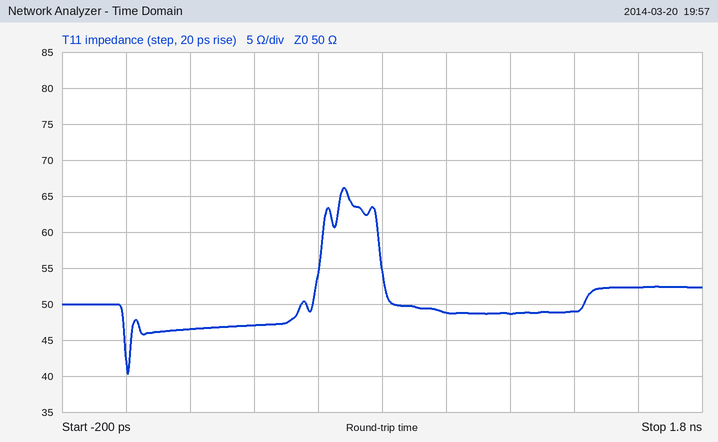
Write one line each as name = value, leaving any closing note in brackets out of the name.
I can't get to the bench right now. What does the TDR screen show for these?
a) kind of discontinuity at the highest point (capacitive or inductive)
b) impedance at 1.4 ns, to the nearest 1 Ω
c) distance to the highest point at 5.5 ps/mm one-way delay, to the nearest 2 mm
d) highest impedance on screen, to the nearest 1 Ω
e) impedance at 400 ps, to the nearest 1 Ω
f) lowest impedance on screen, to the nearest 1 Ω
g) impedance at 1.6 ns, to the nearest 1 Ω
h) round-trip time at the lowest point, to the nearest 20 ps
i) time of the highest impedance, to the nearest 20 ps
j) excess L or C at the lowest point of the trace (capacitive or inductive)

kind of discontinuity at the highest point = inductive
impedance at 1.4 ns, to the nearest 1 Ω = 49 Ω
distance to the highest point at 5.5 ps/mm one-way delay, to the nearest 2 mm = 62 mm
highest impedance on screen, to the nearest 1 Ω = 66 Ω
impedance at 400 ps, to the nearest 1 Ω = 47 Ω
lowest impedance on screen, to the nearest 1 Ω = 40 Ω
impedance at 1.6 ns, to the nearest 1 Ω = 52 Ω
round-trip time at the lowest point, to the nearest 20 ps = 0 ps
time of the highest impedance, to the nearest 20 ps = 680 ps
excess L or C at the lowest point of the trace = capacitive
